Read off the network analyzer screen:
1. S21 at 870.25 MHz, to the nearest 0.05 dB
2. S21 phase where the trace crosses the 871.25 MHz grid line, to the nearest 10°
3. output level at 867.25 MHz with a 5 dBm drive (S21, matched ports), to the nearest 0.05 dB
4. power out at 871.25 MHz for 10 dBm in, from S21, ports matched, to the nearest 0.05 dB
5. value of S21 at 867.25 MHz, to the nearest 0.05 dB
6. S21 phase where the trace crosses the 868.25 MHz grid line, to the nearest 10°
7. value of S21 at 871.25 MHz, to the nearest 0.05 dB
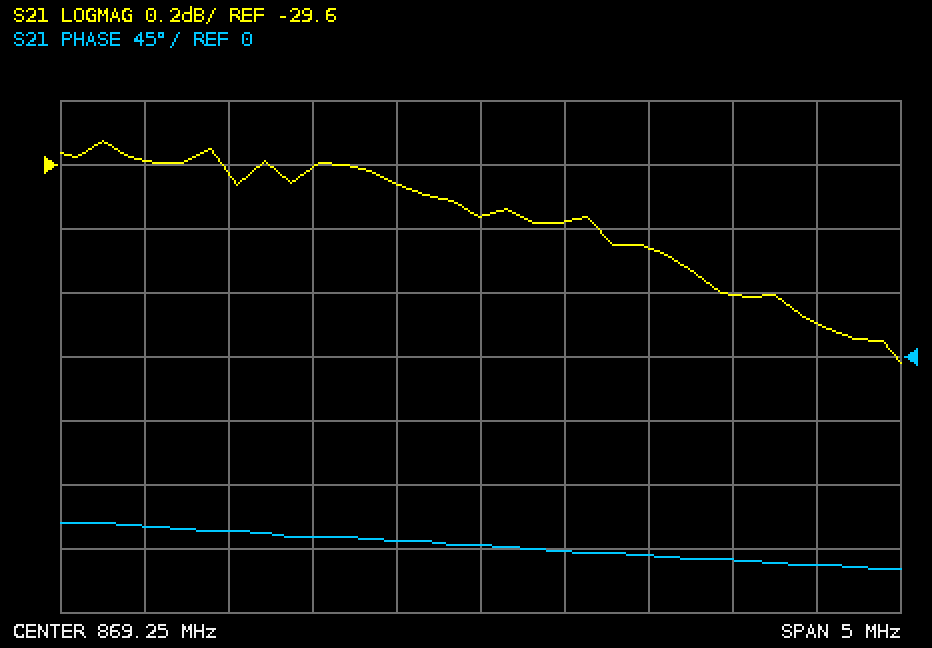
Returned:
-29.85 dB
-150°
-24.60 dBm
-20.10 dBm
-29.60 dB
-130°
-30.10 dB
